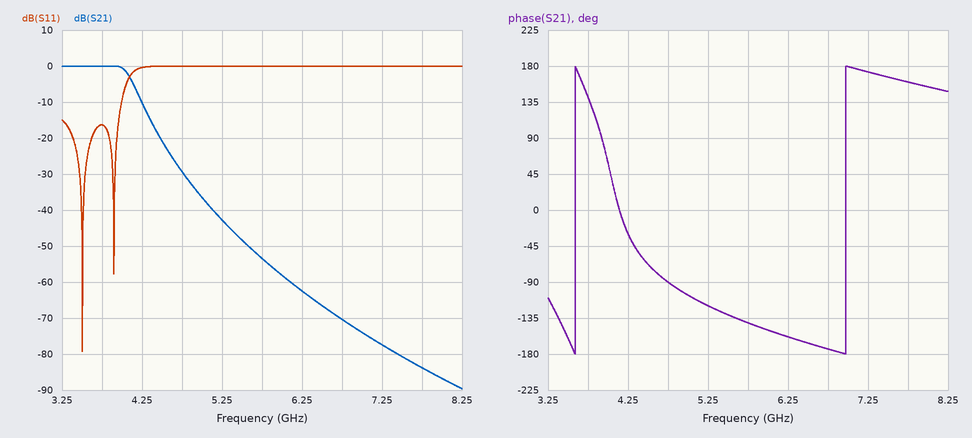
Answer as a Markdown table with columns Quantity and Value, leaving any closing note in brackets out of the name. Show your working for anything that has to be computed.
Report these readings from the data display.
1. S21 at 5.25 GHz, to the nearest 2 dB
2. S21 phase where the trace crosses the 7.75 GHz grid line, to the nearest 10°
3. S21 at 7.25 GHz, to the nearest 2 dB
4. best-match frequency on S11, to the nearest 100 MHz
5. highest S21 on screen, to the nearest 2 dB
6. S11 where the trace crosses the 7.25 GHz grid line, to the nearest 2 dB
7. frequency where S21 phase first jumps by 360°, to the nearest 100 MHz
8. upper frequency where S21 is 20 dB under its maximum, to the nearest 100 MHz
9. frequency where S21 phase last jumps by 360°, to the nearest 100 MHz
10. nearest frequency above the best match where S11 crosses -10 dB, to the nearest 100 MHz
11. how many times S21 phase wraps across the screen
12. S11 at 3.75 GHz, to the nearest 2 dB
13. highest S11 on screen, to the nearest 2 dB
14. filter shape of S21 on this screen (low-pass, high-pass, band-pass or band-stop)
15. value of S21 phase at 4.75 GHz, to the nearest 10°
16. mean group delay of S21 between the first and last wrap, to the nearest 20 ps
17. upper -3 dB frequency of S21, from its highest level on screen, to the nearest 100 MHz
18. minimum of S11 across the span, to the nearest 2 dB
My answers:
| Quantity | Value |
|---|---|
| S21 at 5.25 GHz, to the nearest 2 dB | -42 dB |
| S21 phase where the trace crosses the 7.75 GHz grid line, to the nearest 10° | 160° |
| S21 at 7.25 GHz, to the nearest 2 dB | -78 dB |
| best-match frequency on S11, to the nearest 100 MHz | 3.5 GHz |
| highest S21 on screen, to the nearest 2 dB | 0 dB |
| S11 where the trace crosses the 7.25 GHz grid line, to the nearest 2 dB | 0 dB |
| frequency where S21 phase first jumps by 360°, to the nearest 100 MHz | 3.6 GHz |
| upper frequency where S21 is 20 dB under its maximum, to the nearest 100 MHz | 4.5 GHz |
| frequency where S21 phase last jumps by 360°, to the nearest 100 MHz | 7.0 GHz |
| nearest frequency above the best match where S11 crosses -10 dB, to the nearest 100 MHz | 4.0 GHz |
| how many times S21 phase wraps across the screen | 2 |
| S11 at 3.75 GHz, to the nearest 2 dB | -16 dB |
| highest S11 on screen, to the nearest 2 dB | 0 dB |
| filter shape of S21 on this screen | low-pass |
| value of S21 phase at 4.75 GHz, to the nearest 10° | -90° |
| mean group delay of S21 between the first and last wrap, to the nearest 20 ps | 1 cycle / (7.0 GHz − 3.6 GHz) ≈ 294 ps, so 300 ps to the nearest 20 ps |
| upper -3 dB frequency of S21, from its highest level on screen, to the nearest 100 MHz | 4.1 GHz |
| minimum of S11 across the span, to the nearest 2 dB | -80 dB |
